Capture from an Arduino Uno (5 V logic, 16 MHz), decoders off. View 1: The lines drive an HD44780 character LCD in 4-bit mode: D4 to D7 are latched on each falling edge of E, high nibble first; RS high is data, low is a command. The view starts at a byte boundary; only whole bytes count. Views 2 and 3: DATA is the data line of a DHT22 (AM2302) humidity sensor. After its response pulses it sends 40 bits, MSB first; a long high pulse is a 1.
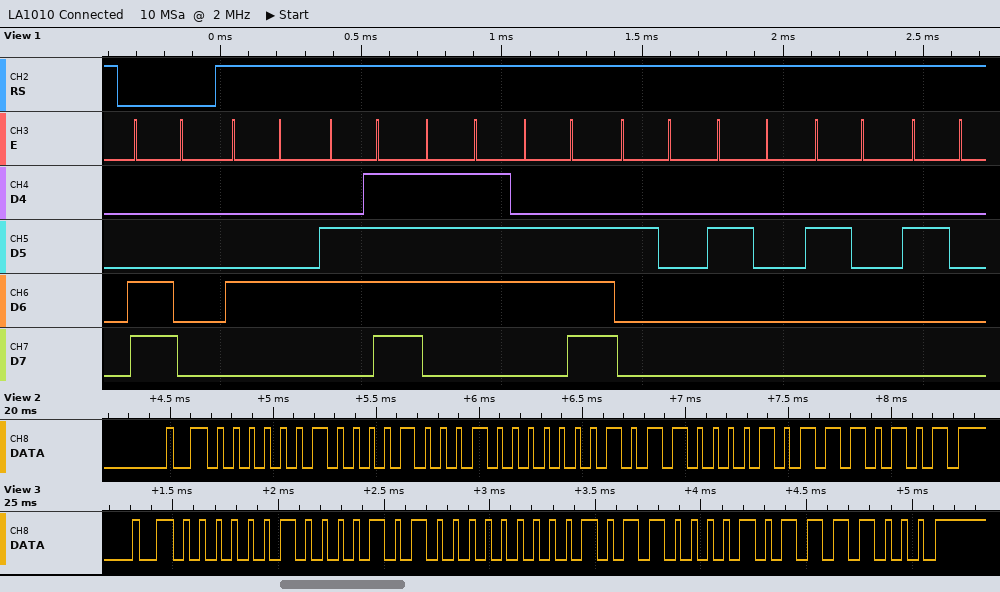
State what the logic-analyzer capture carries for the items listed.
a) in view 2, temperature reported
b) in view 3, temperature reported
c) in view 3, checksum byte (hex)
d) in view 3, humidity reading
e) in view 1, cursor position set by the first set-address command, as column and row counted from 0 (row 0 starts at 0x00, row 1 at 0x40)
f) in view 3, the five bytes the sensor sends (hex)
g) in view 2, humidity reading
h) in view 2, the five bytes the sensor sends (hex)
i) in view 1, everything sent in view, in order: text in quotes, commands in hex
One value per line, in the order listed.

35.3 °C
35.3 °C
0x78
53.2 %
column 0, row 1
02 14 01 61 78
52.9 %
02 11 01 61 75
0xC0 "Down    "
